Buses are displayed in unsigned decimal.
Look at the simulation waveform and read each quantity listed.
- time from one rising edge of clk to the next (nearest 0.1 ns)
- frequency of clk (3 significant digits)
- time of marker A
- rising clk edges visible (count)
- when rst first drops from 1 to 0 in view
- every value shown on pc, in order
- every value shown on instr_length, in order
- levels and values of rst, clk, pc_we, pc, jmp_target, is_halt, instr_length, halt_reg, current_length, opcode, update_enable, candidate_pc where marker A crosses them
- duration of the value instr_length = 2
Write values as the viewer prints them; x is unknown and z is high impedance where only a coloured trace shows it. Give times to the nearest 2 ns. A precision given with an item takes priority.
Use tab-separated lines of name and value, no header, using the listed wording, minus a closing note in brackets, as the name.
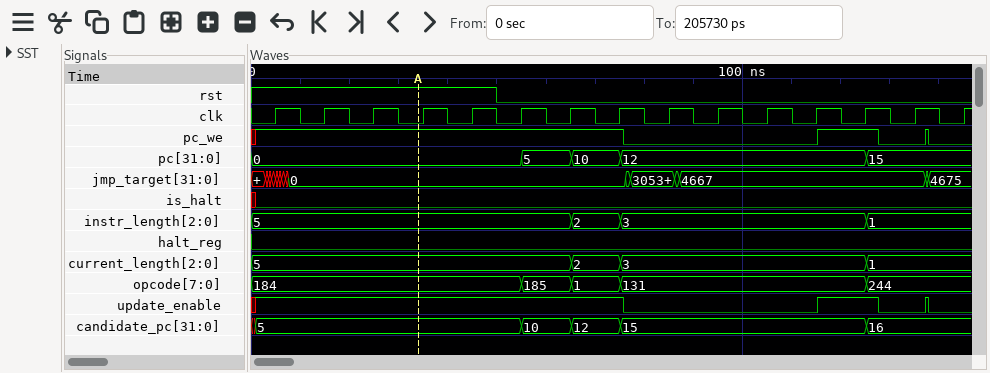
time from one rising edge of clk to the next	10 ns
frequency of clk	100 MHz
time of marker A	34 ns
rising clk edges visible	15
when rst first drops from 1 to 0 in view	50 ns
every value shown on pc, in order	0, 5, 10, 12, 15
every value shown on instr_length, in order	5, 2, 3, 1
levels and values of rst, clk, pc_we, pc, jmp_target, is_halt, instr_length, halt_reg, current_length, opcode, update_enable, candidate_pc where marker A crosses them	rst=1, clk=0, pc_we=1, pc=0, jmp_target=0, is_halt=0, instr_length=5, halt_reg=0, current_length=5, opcode=184, update_enable=1, candidate_pc=5
duration of the value instr_length = 2	10 ns
